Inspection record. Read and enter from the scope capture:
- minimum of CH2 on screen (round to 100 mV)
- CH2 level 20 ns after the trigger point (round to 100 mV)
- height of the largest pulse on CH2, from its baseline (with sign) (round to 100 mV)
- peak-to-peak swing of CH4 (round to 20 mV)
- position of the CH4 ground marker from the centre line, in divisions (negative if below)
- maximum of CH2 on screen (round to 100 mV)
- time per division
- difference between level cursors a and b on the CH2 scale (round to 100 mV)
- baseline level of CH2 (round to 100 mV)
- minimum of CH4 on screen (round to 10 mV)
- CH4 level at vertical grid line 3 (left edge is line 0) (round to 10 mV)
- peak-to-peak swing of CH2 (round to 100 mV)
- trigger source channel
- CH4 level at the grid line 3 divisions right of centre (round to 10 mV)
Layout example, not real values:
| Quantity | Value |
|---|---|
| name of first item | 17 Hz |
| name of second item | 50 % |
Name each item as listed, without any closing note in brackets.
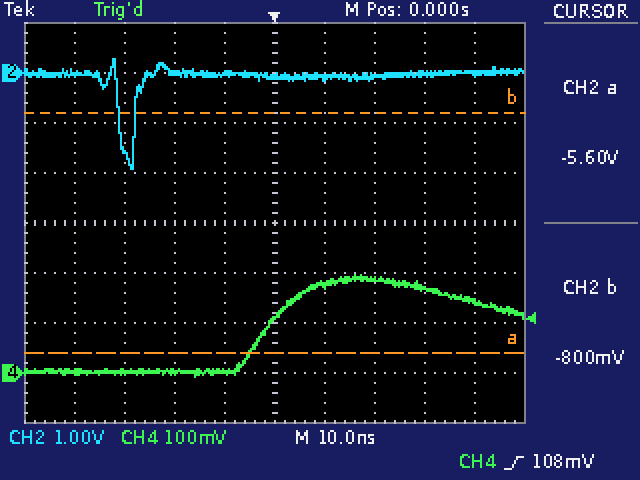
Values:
| Quantity | Value |
|---|---|
| minimum of CH2 on screen | -1.9 V |
| CH2 level 20 ns after the trigger point | -100 mV |
| height of the largest pulse on CH2, from its baseline (with sign) | -1.9 V |
| peak-to-peak swing of CH4 | 200 mV |
| position of the CH4 ground marker from the centre line, in divisions | -3.0 div |
| maximum of CH2 on screen | 300 mV |
| time per division | 10 ns |
| difference between level cursors a and b on the CH2 scale | 4.8 V |
| baseline level of CH2 | 0.0 V |
| minimum of CH4 on screen | -10 mV |
| CH4 level at vertical grid line 3 (left edge is line 0) | 0 mV |
| peak-to-peak swing of CH2 | 2.2 V |
| trigger source channel | CH4 |
| CH4 level at the grid line 3 divisions right of centre | 170 mV |
